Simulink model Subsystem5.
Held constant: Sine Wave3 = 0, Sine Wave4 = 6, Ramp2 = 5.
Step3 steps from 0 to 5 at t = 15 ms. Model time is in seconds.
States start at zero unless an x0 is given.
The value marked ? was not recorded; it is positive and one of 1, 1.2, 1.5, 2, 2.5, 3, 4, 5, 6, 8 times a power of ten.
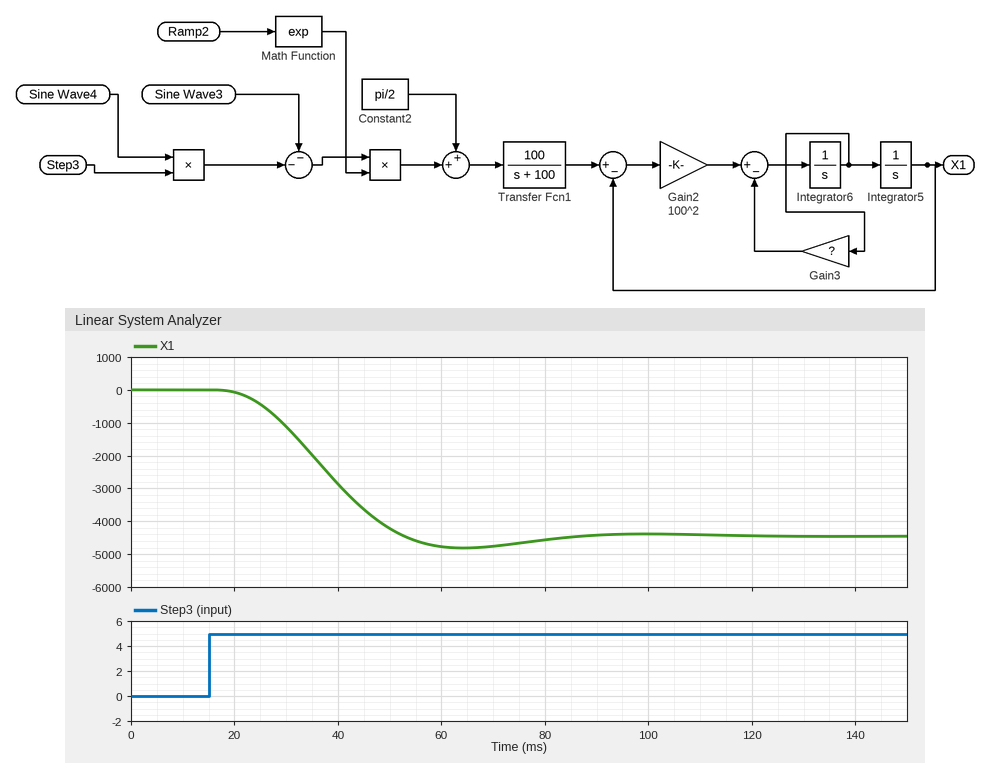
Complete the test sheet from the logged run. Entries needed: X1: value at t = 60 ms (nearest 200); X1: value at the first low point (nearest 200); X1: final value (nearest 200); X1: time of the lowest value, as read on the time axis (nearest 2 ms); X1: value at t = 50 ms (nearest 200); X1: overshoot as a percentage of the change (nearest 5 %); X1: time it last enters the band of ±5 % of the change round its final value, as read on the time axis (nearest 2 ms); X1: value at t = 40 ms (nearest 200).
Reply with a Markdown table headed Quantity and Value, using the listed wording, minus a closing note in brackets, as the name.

| Quantity | Value |
|---|---|
| X1: value at t = 60 ms | -4800 |
| X1: value at the first low point | -4800 |
| X1: final value | -4400 |
| X1: time of the lowest value, as read on the time axis | 64 ms |
| X1: value at t = 50 ms | -4200 |
| X1: overshoot as a percentage of the change | 10 % |
| X1: time it last enters the band of ±5 % of the change round its final value, as read on the time axis | 74 ms |
| X1: value at t = 40 ms | -2800 |
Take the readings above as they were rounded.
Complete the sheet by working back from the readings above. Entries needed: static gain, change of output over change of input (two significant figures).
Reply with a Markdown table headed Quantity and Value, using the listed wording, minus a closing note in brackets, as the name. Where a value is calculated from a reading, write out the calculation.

| Quantity | Value |
|---|---|
| static gain, change of output over change of input | (-4400 - 0) / (5 - 0) = -880 |
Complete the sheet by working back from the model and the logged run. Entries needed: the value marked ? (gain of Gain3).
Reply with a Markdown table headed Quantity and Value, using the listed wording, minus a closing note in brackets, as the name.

| Quantity | Value |
|---|---|
| the value marked ? | 100 |
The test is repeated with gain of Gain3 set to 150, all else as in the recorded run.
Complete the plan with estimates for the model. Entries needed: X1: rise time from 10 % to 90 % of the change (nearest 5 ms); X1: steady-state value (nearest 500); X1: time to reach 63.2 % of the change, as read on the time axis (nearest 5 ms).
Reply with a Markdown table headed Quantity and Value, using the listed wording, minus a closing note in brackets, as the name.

| Quantity | Value |
|---|---|
| X1: rise time from 10 % to 90 % of the change | 30 ms |
| X1: steady-state value | -4500 |
| X1: time to reach 63.2 % of the change, as read on the time axis | 45 ms |
